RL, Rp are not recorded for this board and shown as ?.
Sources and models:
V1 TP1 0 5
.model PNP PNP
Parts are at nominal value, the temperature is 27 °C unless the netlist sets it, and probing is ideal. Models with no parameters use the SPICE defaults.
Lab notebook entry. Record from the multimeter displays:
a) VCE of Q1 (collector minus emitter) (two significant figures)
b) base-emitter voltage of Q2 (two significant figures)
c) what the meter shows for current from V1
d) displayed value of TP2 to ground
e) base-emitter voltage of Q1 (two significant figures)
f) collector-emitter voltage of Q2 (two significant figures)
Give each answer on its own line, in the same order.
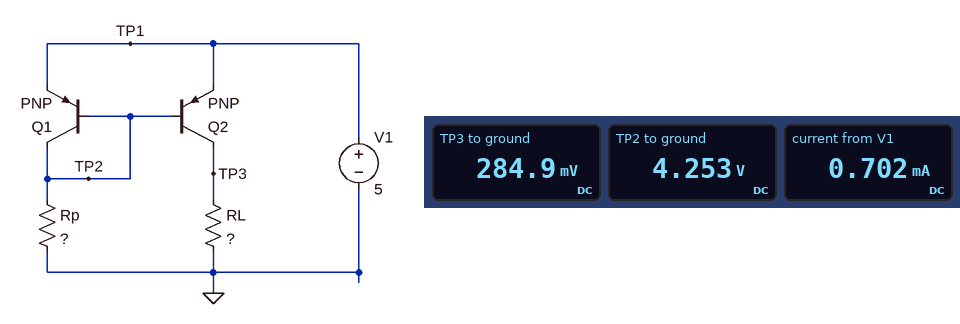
-750 mV
-750 mV
0.702 mA
4.253 V
-750 mV
-4.7 V
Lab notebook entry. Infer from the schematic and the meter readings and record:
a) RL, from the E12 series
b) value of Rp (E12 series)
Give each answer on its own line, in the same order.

820 Ω
12 kΩ
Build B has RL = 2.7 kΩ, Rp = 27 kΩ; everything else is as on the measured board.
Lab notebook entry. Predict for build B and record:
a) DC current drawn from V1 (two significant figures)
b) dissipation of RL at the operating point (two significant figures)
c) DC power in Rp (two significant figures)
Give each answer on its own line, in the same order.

310 µA
65 µW
680 µW
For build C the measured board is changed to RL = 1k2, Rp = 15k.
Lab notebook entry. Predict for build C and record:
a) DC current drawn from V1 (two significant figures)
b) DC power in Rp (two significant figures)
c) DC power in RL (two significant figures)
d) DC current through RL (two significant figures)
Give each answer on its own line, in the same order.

560 µA
1.2 mW
93 µW
280 µA
